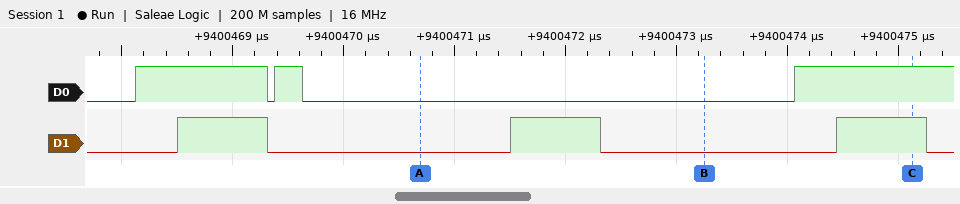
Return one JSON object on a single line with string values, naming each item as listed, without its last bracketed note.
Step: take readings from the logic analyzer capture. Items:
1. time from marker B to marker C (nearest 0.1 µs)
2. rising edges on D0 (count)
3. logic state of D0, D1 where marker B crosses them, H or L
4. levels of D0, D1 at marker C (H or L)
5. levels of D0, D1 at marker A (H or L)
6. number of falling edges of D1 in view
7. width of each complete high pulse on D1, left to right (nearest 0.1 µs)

{"time from marker B to marker C": "1.9 µs", "rising edges on D0": "3", "logic state of D0, D1 where marker B crosses them, H or L": "D0=L, D1=L", "levels of D0, D1 at marker C": "D0=H, D1=H", "levels of D0, D1 at marker A": "D0=L, D1=L", "number of falling edges of D1 in view": "3", "width of each complete high pulse on D1, left to right": "0.8 µs, 0.8 µs, 0.8 µs"}
